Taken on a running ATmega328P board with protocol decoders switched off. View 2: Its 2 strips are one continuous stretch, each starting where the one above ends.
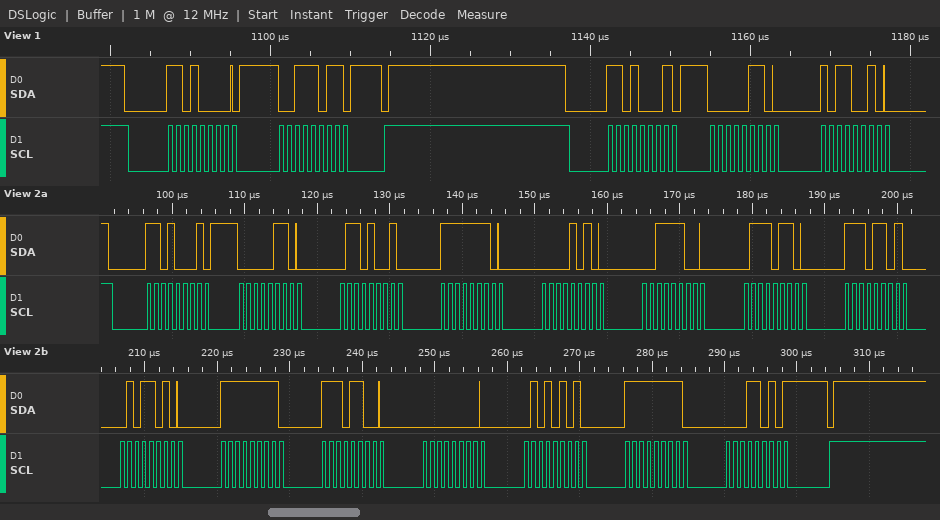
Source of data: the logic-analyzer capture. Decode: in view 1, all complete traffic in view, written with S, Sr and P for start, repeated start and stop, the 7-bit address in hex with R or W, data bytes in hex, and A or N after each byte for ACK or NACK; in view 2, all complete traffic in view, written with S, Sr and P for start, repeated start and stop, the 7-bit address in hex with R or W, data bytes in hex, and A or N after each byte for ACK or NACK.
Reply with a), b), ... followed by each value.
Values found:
a) S 68W A 3B A P S 68R A 06 A B2 A
b) S 68R A 06 A 69 A FE A 0A A 3C A 76 A ED A 5A A FF A EC A 00 A 55 A FF A 1A N P
